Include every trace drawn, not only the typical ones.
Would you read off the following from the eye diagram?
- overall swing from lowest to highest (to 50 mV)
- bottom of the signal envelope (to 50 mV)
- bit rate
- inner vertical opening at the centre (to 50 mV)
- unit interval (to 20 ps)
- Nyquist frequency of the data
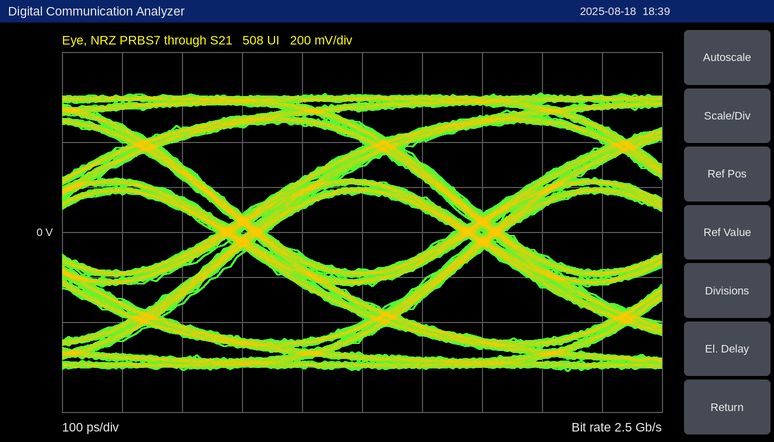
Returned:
1.25 V
-600 mV
2.5 Gb/s
350 mV
400 ps
1.25 GHz
